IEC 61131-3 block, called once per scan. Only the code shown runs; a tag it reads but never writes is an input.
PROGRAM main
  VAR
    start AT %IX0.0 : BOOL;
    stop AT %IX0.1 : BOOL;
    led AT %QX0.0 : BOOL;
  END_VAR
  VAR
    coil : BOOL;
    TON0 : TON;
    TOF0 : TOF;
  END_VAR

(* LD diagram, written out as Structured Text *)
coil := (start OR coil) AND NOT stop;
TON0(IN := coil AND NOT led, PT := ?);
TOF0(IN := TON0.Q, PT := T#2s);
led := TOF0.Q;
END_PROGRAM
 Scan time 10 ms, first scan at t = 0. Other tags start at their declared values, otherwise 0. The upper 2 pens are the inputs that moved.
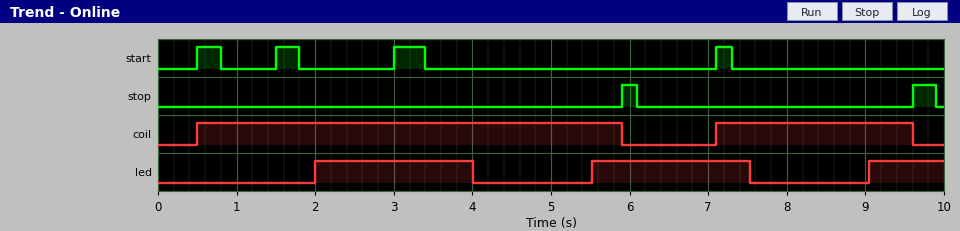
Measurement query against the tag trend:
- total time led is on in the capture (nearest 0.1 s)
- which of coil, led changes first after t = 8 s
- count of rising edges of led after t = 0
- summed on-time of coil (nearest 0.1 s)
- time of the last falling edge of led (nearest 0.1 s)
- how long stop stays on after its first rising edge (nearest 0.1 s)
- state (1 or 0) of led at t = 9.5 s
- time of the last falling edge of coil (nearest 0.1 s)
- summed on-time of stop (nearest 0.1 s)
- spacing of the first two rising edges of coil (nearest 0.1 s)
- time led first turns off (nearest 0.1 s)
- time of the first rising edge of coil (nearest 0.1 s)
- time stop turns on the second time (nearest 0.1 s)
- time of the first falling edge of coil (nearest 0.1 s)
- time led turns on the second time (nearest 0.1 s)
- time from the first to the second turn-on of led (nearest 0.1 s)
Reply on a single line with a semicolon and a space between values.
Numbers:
5.0 s; led; 3; 7.9 s; 7.5 s; 0.2 s; 1; 9.6 s; 0.5 s; 6.6 s; 4.0 s; 0.5 s; 9.6 s; 5.9 s; 5.5 s; 3.5 s
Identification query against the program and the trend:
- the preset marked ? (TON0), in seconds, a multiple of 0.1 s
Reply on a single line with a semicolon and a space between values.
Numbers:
1.5 s
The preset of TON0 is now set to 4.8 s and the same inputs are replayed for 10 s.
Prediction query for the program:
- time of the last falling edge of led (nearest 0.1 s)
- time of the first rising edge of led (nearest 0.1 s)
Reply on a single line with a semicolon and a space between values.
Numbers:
7.3 s; 5.3 s
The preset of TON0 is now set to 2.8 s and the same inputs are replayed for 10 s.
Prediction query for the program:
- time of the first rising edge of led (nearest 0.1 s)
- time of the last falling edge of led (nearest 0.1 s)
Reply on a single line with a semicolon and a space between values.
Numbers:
3.3 s; 5.3 s
